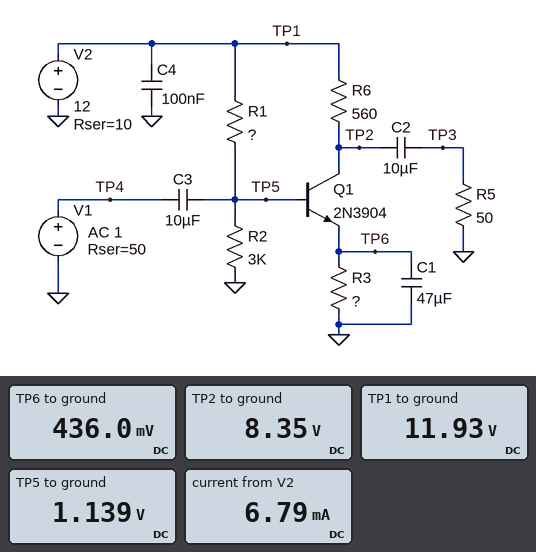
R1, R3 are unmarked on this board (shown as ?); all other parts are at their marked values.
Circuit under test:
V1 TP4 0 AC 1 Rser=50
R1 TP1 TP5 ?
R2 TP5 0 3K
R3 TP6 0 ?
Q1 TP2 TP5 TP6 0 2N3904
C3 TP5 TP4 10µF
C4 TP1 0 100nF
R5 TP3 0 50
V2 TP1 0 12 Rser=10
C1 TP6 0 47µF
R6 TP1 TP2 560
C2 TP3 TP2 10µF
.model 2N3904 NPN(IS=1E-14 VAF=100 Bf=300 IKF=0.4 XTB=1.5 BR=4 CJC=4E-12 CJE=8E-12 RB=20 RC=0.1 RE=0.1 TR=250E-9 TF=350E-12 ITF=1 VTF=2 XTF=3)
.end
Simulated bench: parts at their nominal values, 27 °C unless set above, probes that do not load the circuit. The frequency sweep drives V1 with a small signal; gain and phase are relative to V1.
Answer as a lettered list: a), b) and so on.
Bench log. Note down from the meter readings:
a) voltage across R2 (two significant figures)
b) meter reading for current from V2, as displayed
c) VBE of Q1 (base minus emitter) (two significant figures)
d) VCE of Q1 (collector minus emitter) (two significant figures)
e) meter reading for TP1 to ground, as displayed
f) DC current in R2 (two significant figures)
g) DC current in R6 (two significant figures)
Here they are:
a) 1.1 V
b) 6.79 mA
c) 700 mV
d) 7.9 V
e) 11.93 V
f) 380 µA
g) 6.4 mA
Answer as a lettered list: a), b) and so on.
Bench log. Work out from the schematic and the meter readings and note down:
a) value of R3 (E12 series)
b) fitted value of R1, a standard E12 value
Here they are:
a) 68 Ω
b) 27 kΩ
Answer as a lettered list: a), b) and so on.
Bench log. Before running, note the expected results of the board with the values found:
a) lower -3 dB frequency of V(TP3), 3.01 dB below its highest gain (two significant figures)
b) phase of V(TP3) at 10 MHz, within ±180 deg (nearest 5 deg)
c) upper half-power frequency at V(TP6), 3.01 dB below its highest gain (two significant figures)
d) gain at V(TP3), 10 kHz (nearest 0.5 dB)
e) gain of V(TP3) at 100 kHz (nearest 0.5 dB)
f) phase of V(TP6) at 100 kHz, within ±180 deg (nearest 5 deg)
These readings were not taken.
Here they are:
a) 820 Hz
b) 155 deg
c) 840 Hz
d) 20.0 dB
e) 20.0 dB
f) -90 deg
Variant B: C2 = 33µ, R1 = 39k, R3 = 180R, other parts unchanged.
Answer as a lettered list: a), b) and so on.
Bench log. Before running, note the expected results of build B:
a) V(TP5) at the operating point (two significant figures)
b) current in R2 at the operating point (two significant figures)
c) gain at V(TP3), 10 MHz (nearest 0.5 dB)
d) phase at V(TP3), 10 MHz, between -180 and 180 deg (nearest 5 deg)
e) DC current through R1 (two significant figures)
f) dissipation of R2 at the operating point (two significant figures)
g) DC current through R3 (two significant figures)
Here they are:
a) 850 mV
b) 280 µA
c) 5.0 dB
d) 170 deg
e) 290 µA
f) 240 µW
g) 1.1 mA
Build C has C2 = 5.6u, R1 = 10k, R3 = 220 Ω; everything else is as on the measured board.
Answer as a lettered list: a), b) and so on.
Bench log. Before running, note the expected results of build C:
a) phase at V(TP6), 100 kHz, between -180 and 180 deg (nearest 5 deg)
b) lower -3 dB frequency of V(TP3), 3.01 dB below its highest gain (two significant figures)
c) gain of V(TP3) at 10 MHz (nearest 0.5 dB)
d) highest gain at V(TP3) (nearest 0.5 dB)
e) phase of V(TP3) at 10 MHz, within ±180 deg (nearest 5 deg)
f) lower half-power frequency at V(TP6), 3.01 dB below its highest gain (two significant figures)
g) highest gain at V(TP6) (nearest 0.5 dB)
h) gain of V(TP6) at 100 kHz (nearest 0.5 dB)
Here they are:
a) -90 deg
b) 1.1 kHz
c) 21.0 dB
d) 22.5 dB
e) 145 deg
f) 6.9 Hz
g) -0.5 dB
h) -40.0 dB
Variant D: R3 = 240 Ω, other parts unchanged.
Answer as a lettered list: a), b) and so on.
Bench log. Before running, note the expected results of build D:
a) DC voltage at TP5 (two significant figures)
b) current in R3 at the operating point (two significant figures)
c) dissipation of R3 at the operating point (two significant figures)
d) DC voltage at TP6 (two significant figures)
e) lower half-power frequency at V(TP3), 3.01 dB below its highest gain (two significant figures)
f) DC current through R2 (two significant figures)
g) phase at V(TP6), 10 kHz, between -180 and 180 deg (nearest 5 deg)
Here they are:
a) 1.2 V
b) 2.1 mA
c) 1.1 mW
d) 510 mV
e) 290 Hz
f) 390 µA
g) -90 deg
